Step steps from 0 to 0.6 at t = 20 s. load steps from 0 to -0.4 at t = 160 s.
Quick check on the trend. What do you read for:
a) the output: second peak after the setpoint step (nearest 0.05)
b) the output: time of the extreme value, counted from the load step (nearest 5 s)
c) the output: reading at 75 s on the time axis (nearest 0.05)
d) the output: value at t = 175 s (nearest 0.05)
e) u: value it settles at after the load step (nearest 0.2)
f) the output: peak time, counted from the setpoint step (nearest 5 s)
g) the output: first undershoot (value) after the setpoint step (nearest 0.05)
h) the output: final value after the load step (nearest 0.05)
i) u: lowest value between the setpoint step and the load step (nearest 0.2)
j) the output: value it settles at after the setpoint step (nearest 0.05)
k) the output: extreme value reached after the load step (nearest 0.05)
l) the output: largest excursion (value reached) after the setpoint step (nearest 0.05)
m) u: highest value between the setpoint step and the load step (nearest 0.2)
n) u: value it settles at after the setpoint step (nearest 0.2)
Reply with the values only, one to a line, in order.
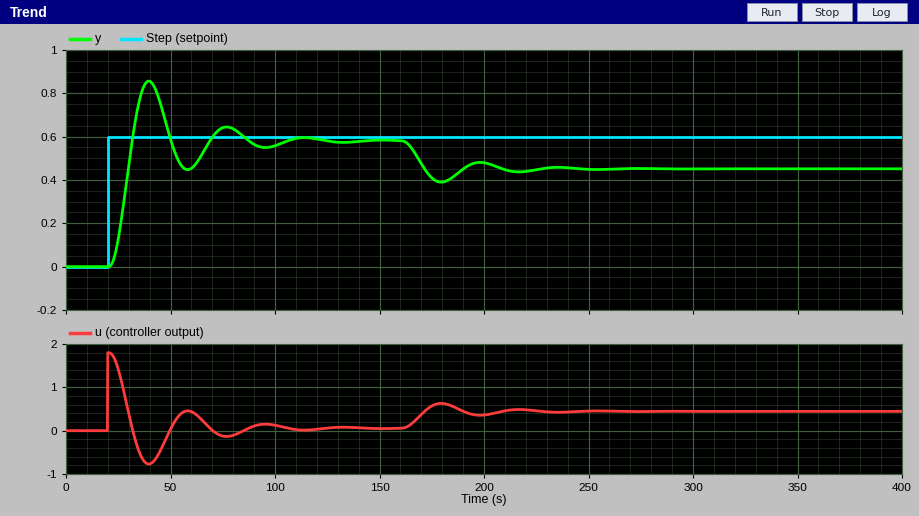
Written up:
0.65
20 s
0.65
0.40
0.4
20 s
0.45
0.45
-0.8
0.60
0.40
0.85
1.8
0.0
